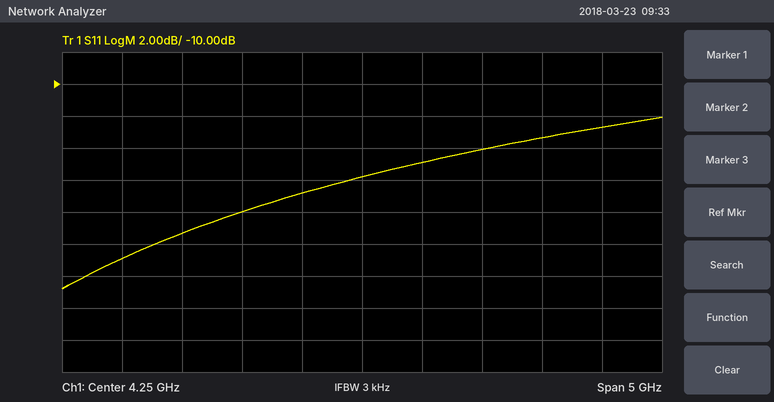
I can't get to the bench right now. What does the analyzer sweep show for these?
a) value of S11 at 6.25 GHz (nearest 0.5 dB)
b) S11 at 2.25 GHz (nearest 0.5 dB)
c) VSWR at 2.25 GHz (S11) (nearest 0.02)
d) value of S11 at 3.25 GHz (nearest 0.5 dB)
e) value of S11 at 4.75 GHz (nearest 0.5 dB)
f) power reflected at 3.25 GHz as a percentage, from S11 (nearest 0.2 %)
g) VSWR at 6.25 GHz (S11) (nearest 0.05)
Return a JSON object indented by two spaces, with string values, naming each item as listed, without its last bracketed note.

{
  "value of S11 at 6.25 GHz": "-12.5 dB",
  "S11 at 2.25 GHz": "-21.0 dB",
  "VSWR at 2.25 GHz (S11)": "1.20",
  "value of S11 at 3.25 GHz": "-18.0 dB",
  "value of S11 at 4.75 GHz": "-15.0 dB",
  "power reflected at 3.25 GHz as a percentage, from S11": "1.6 %",
  "VSWR at 6.25 GHz (S11)": "1.60"
}
